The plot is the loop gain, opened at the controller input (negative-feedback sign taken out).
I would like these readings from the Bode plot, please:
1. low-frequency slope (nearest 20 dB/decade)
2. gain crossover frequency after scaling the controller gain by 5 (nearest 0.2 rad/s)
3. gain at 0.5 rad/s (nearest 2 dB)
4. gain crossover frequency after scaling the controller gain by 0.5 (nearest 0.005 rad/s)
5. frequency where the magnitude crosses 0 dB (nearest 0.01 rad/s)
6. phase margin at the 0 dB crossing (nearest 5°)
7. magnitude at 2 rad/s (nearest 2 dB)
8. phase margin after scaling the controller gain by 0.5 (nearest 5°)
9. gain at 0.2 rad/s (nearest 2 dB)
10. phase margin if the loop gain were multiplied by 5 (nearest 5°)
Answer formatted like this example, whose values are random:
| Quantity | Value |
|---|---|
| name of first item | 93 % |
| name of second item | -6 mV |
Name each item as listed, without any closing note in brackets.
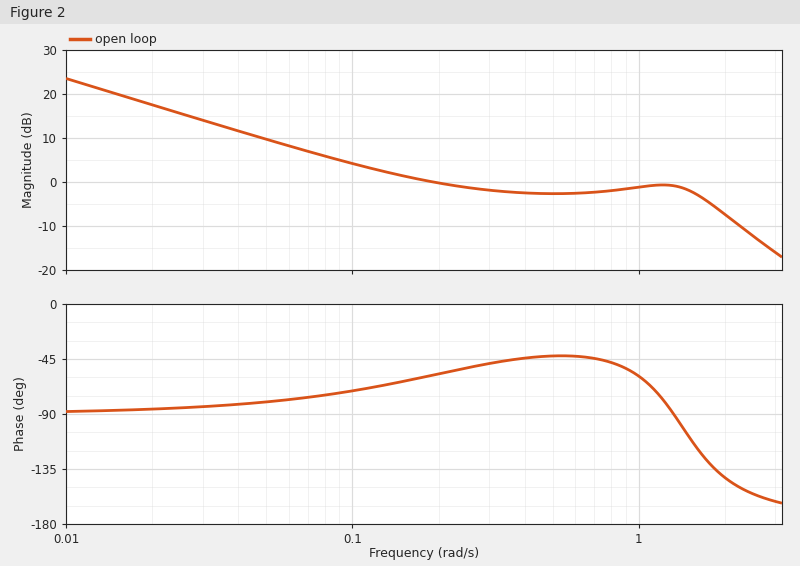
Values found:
| Quantity | Value |
|---|---|
| low-frequency slope | -20 dB/decade |
| gain crossover frequency after scaling the controller gain by 5 | 2.8 rad/s |
| gain at 0.5 rad/s | -2 dB |
| gain crossover frequency after scaling the controller gain by 0.5 | 0.080 rad/s |
| frequency where the magnitude crosses 0 dB | 0.19 rad/s |
| phase margin at the 0 dB crossing | 120° |
| magnitude at 2 rad/s | -8 dB |
| phase margin after scaling the controller gain by 0.5 | 105° |
| gain at 0.2 rad/s | 0 dB |
| phase margin if the loop gain were multiplied by 5 | 20° |
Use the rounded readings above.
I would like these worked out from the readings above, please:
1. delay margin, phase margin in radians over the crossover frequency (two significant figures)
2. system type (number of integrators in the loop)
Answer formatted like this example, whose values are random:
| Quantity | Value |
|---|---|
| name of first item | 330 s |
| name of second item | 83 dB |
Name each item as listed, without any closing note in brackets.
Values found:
| Quantity | Value |
|---|---|
| delay margin, phase margin in radians over the crossover frequency | 11 s |
| system type | 1 |
